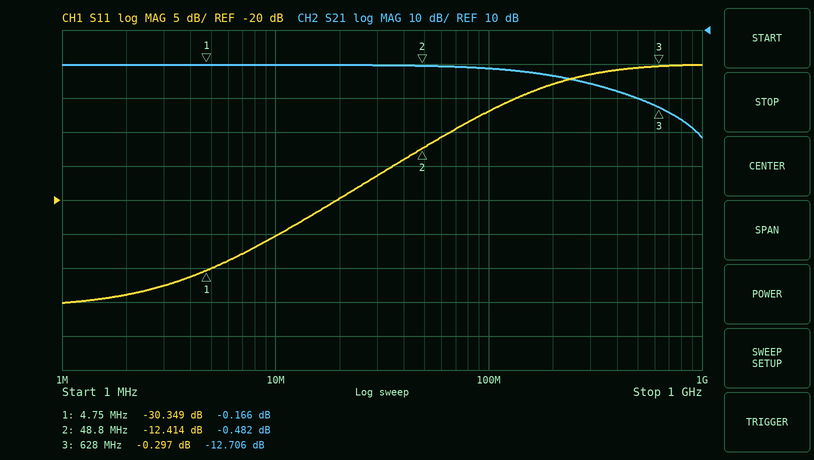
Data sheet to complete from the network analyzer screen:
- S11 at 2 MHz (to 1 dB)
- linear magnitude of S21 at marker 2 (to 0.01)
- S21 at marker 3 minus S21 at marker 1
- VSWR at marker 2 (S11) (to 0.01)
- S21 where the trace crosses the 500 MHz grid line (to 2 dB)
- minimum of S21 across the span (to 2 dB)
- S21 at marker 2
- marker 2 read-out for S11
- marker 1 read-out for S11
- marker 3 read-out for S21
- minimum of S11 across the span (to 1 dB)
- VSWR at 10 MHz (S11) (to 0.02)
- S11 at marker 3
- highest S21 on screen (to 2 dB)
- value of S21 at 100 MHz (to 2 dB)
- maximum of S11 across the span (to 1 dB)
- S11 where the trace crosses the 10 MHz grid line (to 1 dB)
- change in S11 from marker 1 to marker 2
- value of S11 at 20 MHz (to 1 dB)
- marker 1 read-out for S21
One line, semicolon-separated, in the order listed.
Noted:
-34 dB; 0.95; -12.540 dB; 1.63; -10 dB; -22 dB; -0.482 dB; -12.414 dB; -30.349 dB; -12.706 dB; -35 dB; 1.12; -0.297 dB; 0 dB; -2 dB; 0 dB; -25 dB; 17.935 dB; -20 dB; -0.166 dB
